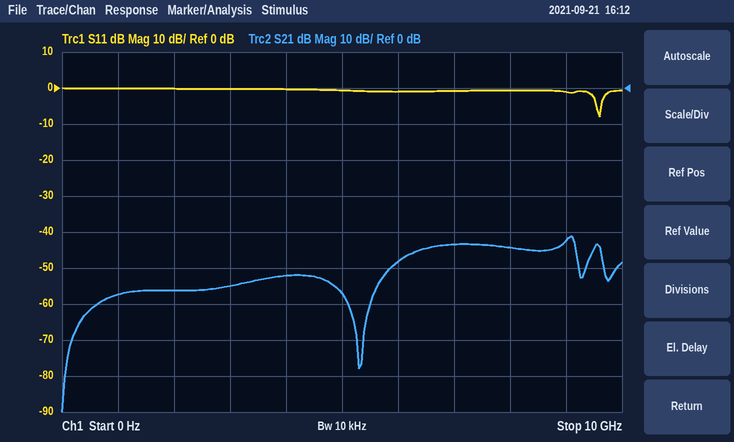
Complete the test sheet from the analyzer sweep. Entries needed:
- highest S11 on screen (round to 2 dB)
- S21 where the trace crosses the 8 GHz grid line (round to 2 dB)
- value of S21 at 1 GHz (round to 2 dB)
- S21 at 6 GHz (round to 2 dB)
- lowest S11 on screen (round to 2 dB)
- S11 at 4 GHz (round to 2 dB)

0 dB
-44 dB
-58 dB
-48 dB
-8 dB
0 dB
